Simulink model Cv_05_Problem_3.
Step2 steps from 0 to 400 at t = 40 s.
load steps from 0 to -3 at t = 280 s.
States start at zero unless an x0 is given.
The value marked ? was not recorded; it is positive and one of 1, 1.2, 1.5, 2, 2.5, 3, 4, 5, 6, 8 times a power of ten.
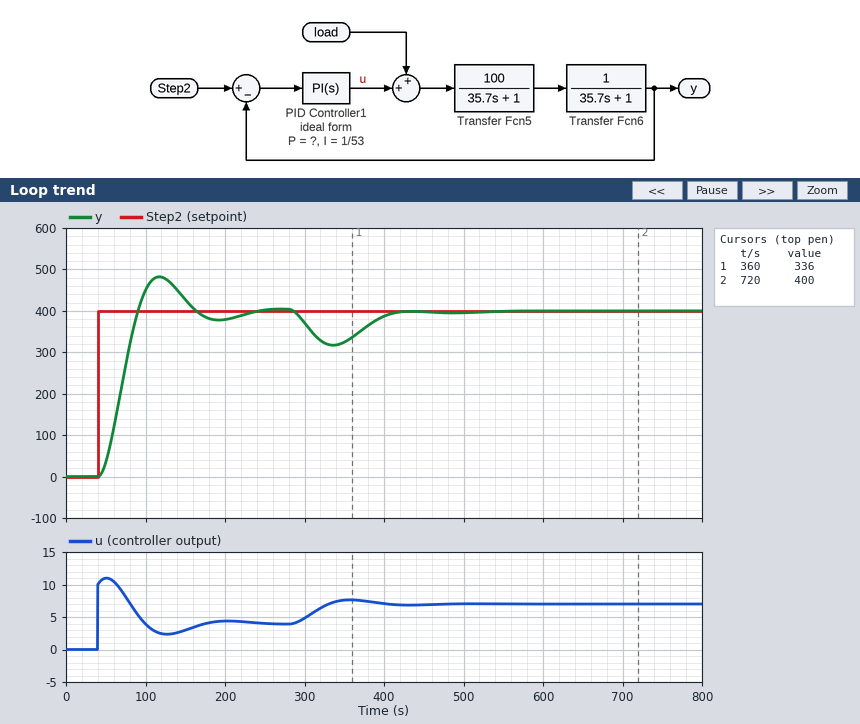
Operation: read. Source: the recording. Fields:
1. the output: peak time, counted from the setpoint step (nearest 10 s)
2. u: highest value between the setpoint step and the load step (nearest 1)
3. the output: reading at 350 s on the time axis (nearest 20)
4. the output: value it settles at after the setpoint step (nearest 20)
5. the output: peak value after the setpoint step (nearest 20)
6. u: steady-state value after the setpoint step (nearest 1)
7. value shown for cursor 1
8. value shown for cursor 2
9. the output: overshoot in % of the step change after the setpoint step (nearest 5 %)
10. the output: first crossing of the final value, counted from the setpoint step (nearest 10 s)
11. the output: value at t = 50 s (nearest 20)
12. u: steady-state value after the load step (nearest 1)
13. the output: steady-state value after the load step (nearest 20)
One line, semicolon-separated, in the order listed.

80 s; 11; 320; 400; 480; 4; 336; 400; 20 %; 50 s; 40; 7; 400
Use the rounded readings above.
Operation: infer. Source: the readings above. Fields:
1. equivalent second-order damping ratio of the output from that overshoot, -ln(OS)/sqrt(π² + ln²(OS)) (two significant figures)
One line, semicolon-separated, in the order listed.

0.46
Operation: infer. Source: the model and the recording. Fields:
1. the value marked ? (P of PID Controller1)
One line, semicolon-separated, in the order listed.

0.025
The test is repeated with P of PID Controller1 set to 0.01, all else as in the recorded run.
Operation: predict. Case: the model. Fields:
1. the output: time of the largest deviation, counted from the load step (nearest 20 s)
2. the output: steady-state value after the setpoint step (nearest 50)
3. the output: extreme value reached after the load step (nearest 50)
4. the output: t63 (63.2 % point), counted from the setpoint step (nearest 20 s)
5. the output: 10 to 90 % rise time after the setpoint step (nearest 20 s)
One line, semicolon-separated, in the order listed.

80 s; 400; 250; 60 s; 80 s
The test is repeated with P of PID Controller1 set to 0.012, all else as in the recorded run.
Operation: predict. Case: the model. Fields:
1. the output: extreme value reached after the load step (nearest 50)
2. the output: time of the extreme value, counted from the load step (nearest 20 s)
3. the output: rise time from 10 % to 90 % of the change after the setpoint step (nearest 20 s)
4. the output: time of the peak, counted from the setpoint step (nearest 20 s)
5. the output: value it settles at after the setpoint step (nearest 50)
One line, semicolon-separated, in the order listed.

300; 80 s; 60 s; 120 s; 400
